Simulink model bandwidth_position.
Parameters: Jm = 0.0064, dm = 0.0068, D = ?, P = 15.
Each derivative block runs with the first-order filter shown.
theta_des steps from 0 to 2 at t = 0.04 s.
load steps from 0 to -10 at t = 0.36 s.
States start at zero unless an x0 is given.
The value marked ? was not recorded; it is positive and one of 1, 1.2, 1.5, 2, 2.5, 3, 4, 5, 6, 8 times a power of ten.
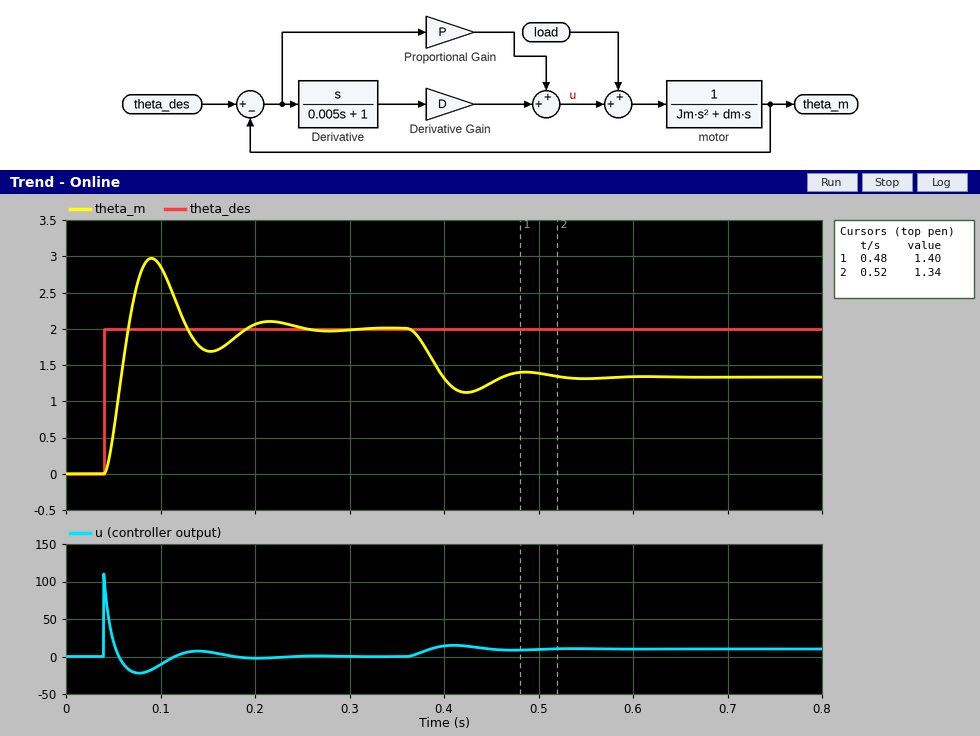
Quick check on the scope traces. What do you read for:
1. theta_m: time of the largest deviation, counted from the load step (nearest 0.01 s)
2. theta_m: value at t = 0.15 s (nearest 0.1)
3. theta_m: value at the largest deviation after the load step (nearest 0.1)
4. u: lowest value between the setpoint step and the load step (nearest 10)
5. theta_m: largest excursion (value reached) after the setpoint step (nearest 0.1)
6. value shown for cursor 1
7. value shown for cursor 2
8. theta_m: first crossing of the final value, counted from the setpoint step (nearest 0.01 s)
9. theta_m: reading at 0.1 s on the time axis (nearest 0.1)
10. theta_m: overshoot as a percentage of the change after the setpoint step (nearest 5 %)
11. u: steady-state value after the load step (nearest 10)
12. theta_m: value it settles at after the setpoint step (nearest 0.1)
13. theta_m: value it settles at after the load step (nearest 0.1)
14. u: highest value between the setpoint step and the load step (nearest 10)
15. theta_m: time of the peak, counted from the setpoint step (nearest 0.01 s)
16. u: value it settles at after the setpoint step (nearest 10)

0.06 s
1.7
1.1
-20
3.0
1.40
1.34
0.03 s
2.9
50 %
10
2.0
1.3
110
0.05 s
0
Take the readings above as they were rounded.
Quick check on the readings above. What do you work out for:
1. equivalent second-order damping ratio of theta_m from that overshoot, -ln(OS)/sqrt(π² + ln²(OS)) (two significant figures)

0.22
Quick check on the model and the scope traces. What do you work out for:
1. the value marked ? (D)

0.2
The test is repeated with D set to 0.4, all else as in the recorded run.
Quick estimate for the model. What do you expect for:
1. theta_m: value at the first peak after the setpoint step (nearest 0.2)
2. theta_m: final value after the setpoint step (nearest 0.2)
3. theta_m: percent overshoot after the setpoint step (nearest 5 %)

2.6
2.0
30 %
